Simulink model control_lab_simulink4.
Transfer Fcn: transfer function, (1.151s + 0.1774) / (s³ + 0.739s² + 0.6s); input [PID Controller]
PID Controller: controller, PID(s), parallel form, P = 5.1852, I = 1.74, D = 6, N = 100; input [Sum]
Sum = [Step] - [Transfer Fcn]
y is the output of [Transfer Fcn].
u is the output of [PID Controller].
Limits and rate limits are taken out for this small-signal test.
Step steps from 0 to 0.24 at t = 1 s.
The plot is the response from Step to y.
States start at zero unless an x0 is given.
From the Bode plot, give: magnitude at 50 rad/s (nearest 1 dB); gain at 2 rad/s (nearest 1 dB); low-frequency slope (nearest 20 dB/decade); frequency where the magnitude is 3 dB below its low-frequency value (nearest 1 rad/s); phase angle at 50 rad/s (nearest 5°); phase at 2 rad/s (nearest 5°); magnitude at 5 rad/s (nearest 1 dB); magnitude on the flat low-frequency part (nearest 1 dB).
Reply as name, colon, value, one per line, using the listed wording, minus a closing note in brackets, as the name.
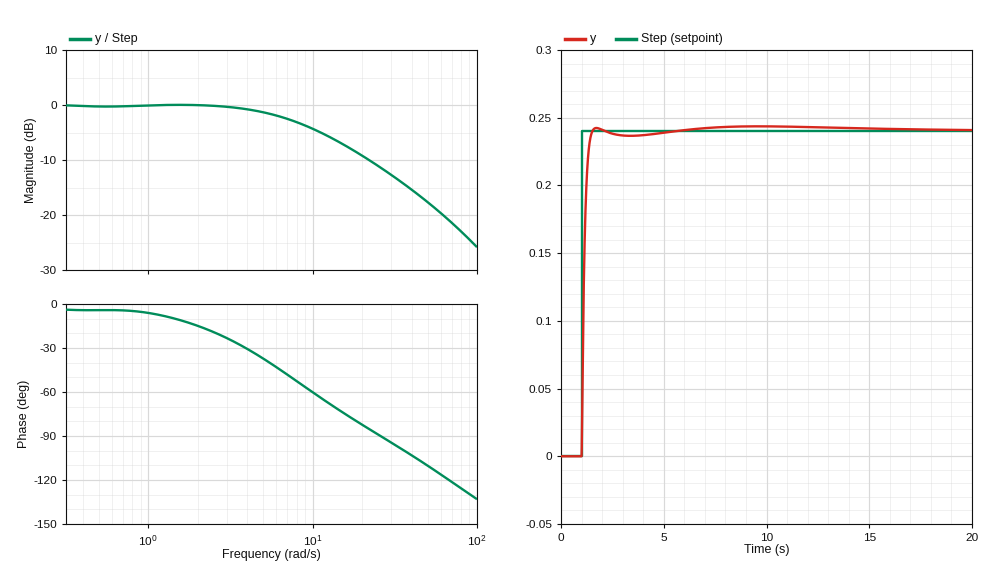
magnitude at 50 rad/s: -18 dB
gain at 2 rad/s: 0 dB
low-frequency slope: 0 dB/decade
frequency where the magnitude is 3 dB below its low-frequency value: 8 rad/s
phase angle at 50 rad/s: -110°
phase at 2 rad/s: -15°
magnitude at 5 rad/s: -1 dB
magnitude on the flat low-frequency part: 0 dB
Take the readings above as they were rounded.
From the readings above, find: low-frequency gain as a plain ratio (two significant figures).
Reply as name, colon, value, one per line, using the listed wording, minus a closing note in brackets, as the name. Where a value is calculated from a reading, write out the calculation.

low-frequency gain as a plain ratio: 10^(0 / 20) = 1.0
